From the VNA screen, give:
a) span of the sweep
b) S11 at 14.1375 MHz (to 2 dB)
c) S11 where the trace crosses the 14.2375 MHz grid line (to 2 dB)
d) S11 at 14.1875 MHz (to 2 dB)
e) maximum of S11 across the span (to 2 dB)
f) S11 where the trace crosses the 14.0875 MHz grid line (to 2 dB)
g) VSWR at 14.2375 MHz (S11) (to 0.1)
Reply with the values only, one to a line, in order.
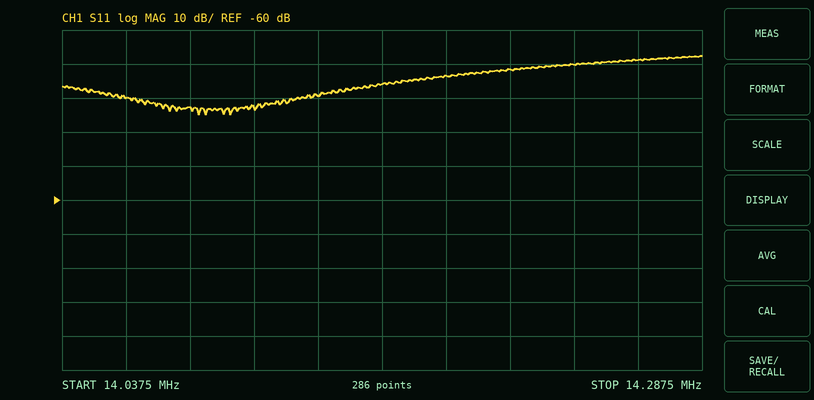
250 kHz
-30 dB
-20 dB
-24 dB
-18 dB
-32 dB
1.2
